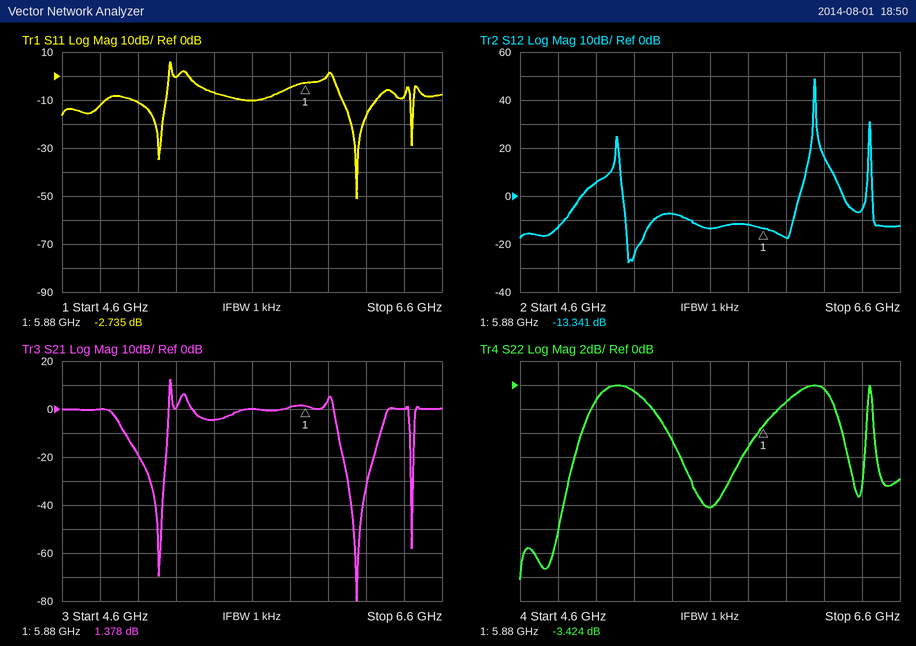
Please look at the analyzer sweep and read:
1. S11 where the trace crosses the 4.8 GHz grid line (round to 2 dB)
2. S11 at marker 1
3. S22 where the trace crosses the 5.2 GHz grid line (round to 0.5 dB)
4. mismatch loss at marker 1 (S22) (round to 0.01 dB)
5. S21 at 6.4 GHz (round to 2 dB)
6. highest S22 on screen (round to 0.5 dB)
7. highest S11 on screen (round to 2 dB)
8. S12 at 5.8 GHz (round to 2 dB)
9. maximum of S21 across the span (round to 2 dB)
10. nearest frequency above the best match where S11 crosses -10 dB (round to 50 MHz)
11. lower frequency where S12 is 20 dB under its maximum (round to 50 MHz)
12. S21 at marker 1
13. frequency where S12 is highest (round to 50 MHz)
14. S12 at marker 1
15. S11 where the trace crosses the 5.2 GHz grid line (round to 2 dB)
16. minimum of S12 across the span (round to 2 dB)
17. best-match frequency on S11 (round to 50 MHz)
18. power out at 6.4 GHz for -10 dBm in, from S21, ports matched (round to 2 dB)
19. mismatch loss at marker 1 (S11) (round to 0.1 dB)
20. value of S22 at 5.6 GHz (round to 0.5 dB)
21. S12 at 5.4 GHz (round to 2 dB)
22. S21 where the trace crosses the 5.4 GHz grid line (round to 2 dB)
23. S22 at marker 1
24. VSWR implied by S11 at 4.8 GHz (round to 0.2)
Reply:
-12 dB
-2.735 dB
-0.5 dB
2.63 dB
0 dB
0.0 dB
6 dB
-12 dB
12 dB
6.25 GHz
6.15 GHz
1.378 dB
6.15 GHz
-13.341 dB
0 dB
-28 dB
6.15 GHz
-10 dBm
3.3 dB
-10.0 dB
-8 dB
-4 dB
-3.424 dB
1.6
